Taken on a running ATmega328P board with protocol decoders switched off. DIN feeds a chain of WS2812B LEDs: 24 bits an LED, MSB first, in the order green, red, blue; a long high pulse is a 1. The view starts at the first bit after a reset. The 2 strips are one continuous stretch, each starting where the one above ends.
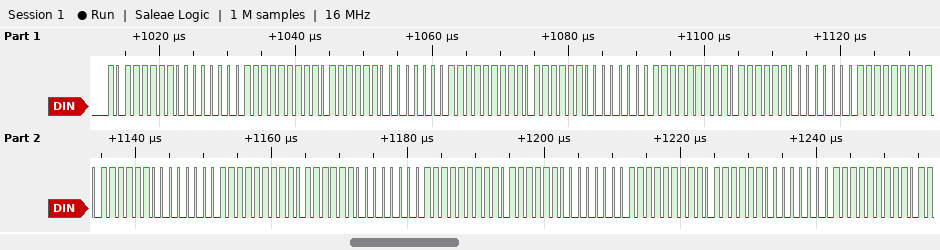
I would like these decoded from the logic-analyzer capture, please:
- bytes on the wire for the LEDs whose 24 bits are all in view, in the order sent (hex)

BF 00 FF BF 00 FF BF 00 FF BF 00 FF BF 00 FF BF 00 FF BF 00 FF BF 00 FF
